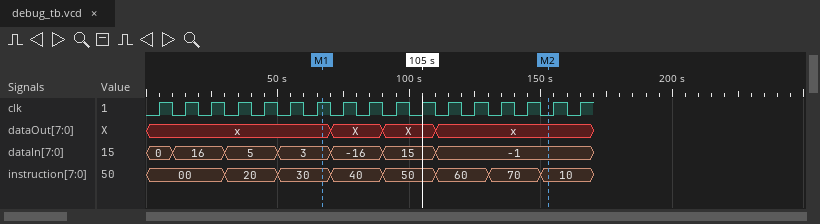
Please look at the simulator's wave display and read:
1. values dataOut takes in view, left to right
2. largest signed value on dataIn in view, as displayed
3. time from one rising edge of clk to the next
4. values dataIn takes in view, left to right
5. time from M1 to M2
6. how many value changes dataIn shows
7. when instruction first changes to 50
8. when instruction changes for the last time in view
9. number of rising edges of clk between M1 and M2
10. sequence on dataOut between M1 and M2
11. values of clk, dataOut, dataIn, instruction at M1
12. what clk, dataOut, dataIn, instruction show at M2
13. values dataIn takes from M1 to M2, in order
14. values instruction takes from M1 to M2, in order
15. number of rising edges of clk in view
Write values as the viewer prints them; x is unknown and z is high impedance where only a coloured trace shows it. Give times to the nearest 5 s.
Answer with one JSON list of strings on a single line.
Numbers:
["x, X, X, x", "16", "10 s", "0, 16, 5, 3, -16, 15, -1", "85 s", "6", "90 s", "150 s", "8", "x, X, X, x", "clk=1, dataOut=x, dataIn=3, instruction=30", "clk=0, dataOut=x, dataIn=-1, instruction=10", "3, -16, 15, -1", "30, 40, 50, 60, 70, 10", "17"]
